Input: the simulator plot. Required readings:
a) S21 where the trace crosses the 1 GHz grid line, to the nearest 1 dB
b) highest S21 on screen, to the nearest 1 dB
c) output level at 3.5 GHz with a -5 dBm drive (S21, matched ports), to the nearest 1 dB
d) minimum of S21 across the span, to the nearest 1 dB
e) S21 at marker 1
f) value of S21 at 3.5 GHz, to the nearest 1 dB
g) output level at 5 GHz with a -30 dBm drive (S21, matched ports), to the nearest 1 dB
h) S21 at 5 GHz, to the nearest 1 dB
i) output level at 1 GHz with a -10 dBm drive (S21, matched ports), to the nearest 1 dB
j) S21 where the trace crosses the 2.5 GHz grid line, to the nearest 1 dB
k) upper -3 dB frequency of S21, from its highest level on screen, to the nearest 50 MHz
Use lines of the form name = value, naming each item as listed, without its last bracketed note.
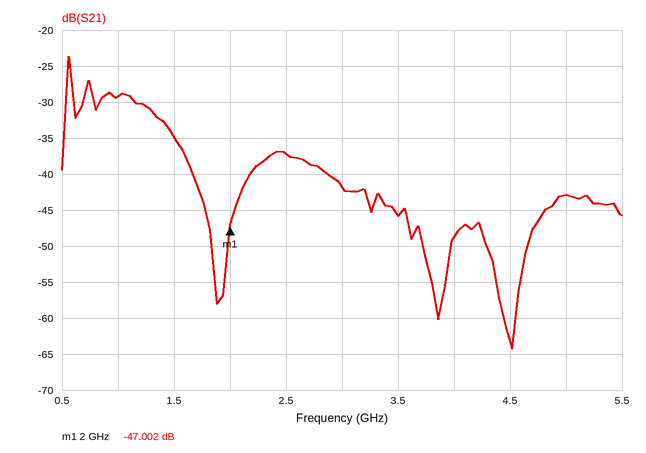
S21 where the trace crosses the 1 GHz grid line, to the nearest 1 dB = -29 dB
highest S21 on screen, to the nearest 1 dB = -24 dB
output level at 3.5 GHz with a -5 dBm drive (S21, matched ports), to the nearest 1 dB = -51 dBm
minimum of S21 across the span, to the nearest 1 dB = -64 dB
S21 at marker 1 = -47.002 dB
value of S21 at 3.5 GHz, to the nearest 1 dB = -46 dB
output level at 5 GHz with a -30 dBm drive (S21, matched ports), to the nearest 1 dB = -73 dBm
S21 at 5 GHz, to the nearest 1 dB = -43 dB
output level at 1 GHz with a -10 dBm drive (S21, matched ports), to the nearest 1 dB = -39 dBm
S21 where the trace crosses the 2.5 GHz grid line, to the nearest 1 dB = -37 dB
upper -3 dB frequency of S21, from its highest level on screen, to the nearest 50 MHz = 600 MHz
